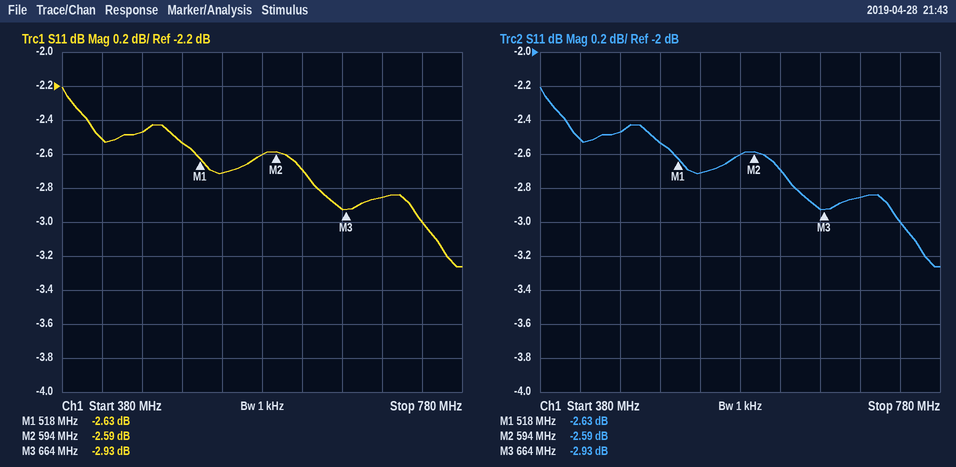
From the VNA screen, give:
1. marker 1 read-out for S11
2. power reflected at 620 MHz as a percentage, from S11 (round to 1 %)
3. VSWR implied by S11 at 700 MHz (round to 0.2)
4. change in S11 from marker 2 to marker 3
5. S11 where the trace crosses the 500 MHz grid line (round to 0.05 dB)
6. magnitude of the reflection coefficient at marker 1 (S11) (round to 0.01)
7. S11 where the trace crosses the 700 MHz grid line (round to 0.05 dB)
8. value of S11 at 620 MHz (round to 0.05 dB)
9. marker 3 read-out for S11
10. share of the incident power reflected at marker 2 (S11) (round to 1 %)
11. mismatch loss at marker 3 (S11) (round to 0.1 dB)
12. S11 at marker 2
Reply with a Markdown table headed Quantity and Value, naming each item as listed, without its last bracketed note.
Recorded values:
| Quantity | Value |
|---|---|
| marker 1 read-out for S11 | -2.63 dB |
| power reflected at 620 MHz as a percentage, from S11 | 54 % |
| VSWR implied by S11 at 700 MHz | 6.2 |
| change in S11 from marker 2 to marker 3 | -0.34 dB |
| S11 where the trace crosses the 500 MHz grid line | -2.55 dB |
| magnitude of the reflection coefficient at marker 1 (S11) | 0.74 |
| S11 where the trace crosses the 700 MHz grid line | -2.85 dB |
| value of S11 at 620 MHz | -2.70 dB |
| marker 3 read-out for S11 | -2.93 dB |
| share of the incident power reflected at marker 2 (S11) | 55 % |
| mismatch loss at marker 3 (S11) | 3.1 dB |
| S11 at marker 2 | -2.59 dB |
